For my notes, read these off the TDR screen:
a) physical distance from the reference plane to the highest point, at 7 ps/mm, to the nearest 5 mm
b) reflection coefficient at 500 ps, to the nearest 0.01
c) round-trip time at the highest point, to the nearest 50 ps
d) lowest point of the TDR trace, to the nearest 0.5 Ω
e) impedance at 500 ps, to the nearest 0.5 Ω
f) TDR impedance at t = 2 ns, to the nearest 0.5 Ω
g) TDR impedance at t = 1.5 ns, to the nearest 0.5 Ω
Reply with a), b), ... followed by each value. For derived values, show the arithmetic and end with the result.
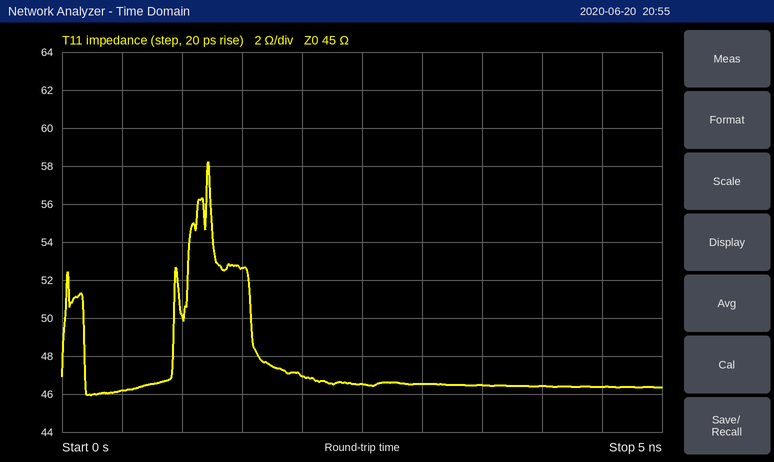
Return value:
a) 1.20 ns / 2 / 7 ps/mm ≈ 85.7 mm, so 85 mm to the nearest 5 mm
b) (46 − 45)/(46 + 45) ≈ +0.01
c) 1.20 ns
d) 46.0 Ω
e) 46.0 Ω
f) 47.0 Ω
g) 52.5 Ω
